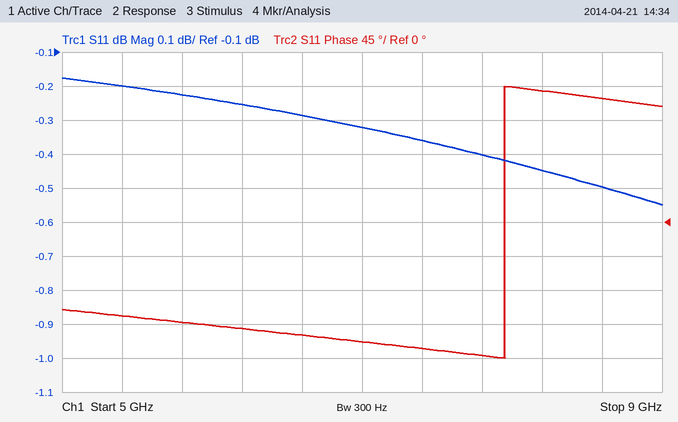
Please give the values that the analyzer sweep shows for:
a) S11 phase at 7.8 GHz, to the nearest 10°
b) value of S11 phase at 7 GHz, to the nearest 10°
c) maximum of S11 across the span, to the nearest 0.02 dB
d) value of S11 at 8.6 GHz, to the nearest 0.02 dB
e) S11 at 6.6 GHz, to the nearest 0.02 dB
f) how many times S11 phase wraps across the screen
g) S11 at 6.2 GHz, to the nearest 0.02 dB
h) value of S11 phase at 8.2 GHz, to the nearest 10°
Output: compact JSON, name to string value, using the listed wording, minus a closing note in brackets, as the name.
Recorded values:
{"S11 phase at 7.8 GHz, to the nearest 10°": "-180°", "value of S11 phase at 7 GHz, to the nearest 10°": "-160°", "maximum of S11 across the span, to the nearest 0.02 dB": "-0.18 dB", "value of S11 at 8.6 GHz, to the nearest 0.02 dB": "-0.50 dB", "S11 at 6.6 GHz, to the nearest 0.02 dB": "-0.28 dB", "how many times S11 phase wraps across the screen": "1", "S11 at 6.2 GHz, to the nearest 0.02 dB": "-0.26 dB", "value of S11 phase at 8.2 GHz, to the nearest 10°": "170°"}
